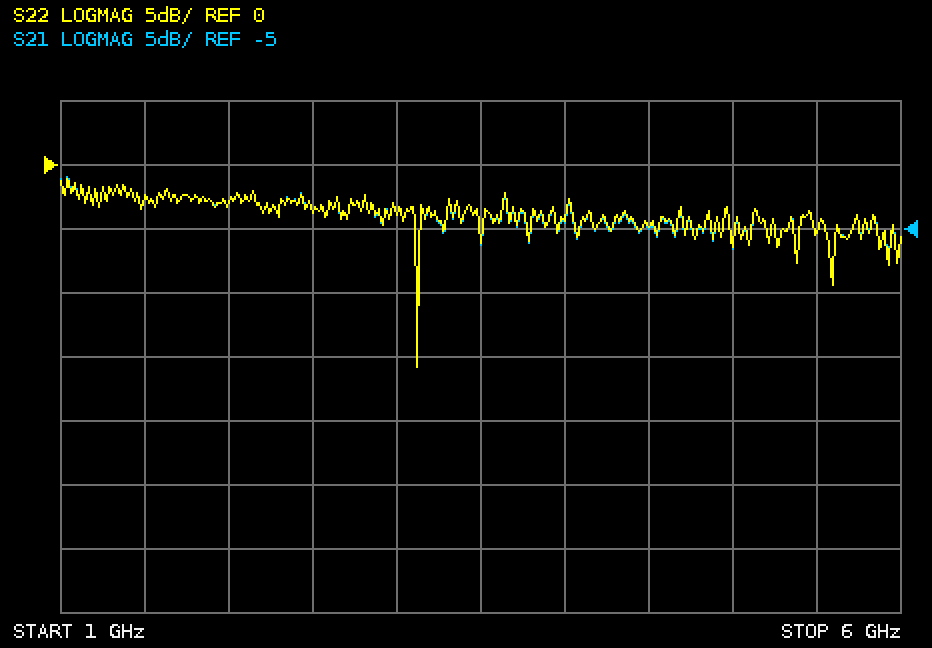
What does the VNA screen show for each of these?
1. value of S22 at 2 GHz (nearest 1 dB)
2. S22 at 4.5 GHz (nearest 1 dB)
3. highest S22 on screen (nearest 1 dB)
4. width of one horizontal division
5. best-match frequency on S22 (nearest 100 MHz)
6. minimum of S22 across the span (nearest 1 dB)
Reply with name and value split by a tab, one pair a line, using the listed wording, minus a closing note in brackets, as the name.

value of S22 at 2 GHz	-3 dB
S22 at 4.5 GHz	-5 dB
highest S22 on screen	-1 dB
width of one horizontal division	500 MHz
best-match frequency on S22	3.1 GHz
minimum of S22 across the span	-16 dB
